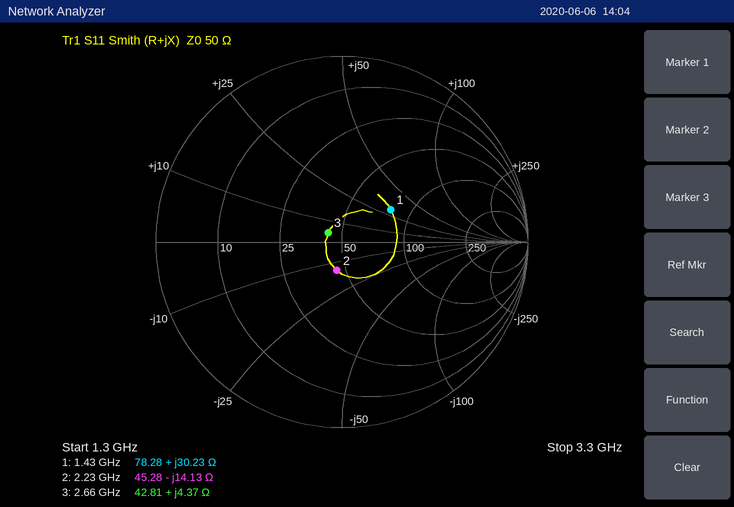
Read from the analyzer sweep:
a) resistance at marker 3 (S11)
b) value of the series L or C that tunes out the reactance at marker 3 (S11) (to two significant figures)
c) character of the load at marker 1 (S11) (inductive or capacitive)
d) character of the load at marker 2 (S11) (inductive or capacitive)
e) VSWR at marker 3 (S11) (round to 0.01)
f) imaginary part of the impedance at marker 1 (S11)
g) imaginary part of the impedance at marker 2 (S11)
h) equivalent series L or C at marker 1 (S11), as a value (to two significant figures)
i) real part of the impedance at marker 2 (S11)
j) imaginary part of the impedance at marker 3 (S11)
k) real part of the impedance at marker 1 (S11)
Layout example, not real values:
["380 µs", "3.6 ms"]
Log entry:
["42.81 Ω", "14 pF", "inductive", "capacitive", "1.20", "+30.23 Ω", "-14.13 Ω", "3.4 nH", "45.28 Ω", "+4.37 Ω", "78.28 Ω"]
